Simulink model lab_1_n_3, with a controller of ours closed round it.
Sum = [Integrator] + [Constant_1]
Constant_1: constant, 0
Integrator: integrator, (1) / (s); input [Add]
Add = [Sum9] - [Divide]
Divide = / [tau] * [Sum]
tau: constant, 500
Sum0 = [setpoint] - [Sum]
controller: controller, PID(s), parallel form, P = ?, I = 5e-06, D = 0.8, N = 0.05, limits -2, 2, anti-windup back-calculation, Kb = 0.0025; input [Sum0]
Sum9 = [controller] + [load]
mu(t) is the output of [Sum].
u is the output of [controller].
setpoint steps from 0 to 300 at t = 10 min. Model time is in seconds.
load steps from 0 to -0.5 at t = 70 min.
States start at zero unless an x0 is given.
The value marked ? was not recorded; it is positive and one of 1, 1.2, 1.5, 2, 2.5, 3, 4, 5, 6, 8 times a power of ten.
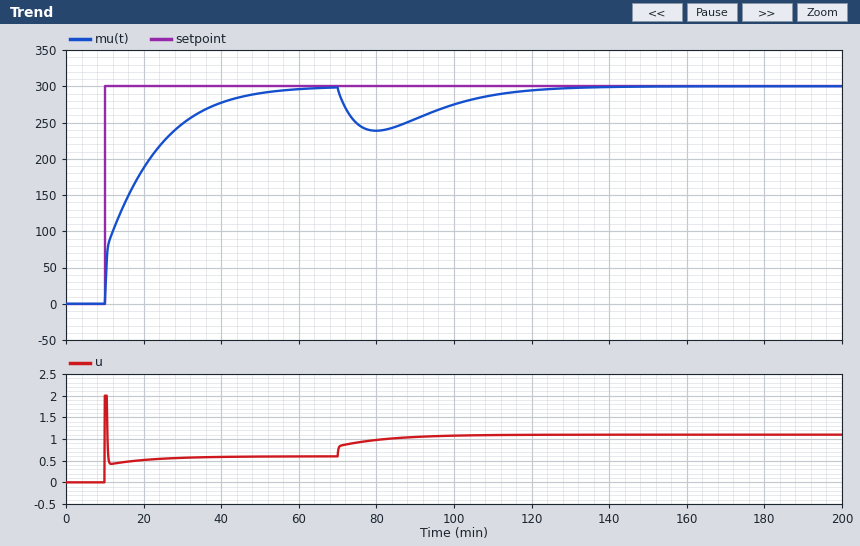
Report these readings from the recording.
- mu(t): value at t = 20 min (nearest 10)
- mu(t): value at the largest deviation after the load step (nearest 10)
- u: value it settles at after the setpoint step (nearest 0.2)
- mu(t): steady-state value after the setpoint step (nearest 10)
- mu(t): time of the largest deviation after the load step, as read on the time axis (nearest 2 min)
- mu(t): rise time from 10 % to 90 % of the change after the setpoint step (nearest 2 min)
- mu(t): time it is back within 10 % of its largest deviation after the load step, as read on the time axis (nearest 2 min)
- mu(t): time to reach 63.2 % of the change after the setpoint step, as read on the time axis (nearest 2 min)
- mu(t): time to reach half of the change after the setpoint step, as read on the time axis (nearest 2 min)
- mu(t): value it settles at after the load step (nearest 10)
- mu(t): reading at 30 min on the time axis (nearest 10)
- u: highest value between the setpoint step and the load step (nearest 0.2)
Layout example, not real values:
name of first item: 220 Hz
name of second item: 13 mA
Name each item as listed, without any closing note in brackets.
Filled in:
mu(t): value at t = 20 min: 190
mu(t): value at the largest deviation after the load step: 240
u: value it settles at after the setpoint step: 0.6
mu(t): steady-state value after the setpoint step: 300
mu(t): time of the largest deviation after the load step, as read on the time axis: 80 min
mu(t): rise time from 10 % to 90 % of the change after the setpoint step: 26 min
mu(t): time it is back within 10 % of its largest deviation after the load step, as read on the time axis: 120 min
mu(t): time to reach 63.2 % of the change after the setpoint step, as read on the time axis: 20 min
mu(t): time to reach half of the change after the setpoint step, as read on the time axis: 16 min
mu(t): value it settles at after the load step: 300
mu(t): reading at 30 min on the time axis: 250
u: highest value between the setpoint step and the load step: 2.0
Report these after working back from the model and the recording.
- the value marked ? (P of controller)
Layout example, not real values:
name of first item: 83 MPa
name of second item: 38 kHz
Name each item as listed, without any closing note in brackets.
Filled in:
the value marked ?: 0.004
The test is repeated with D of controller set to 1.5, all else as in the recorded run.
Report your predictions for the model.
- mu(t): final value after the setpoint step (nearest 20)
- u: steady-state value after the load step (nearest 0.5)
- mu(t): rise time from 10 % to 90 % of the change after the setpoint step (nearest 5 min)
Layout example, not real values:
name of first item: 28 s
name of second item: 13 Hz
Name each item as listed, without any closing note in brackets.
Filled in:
mu(t): final value after the setpoint step: 300
u: steady-state value after the load step: 1.0
mu(t): rise time from 10 % to 90 % of the change after the setpoint step: 35 min
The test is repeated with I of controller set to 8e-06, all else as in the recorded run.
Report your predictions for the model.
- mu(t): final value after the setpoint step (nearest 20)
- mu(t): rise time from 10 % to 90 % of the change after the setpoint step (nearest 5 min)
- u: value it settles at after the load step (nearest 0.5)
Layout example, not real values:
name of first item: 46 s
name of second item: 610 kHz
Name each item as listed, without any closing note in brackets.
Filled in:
mu(t): final value after the setpoint step: 300
mu(t): rise time from 10 % to 90 % of the change after the setpoint step: 15 min
u: value it settles at after the load step: 1.0
